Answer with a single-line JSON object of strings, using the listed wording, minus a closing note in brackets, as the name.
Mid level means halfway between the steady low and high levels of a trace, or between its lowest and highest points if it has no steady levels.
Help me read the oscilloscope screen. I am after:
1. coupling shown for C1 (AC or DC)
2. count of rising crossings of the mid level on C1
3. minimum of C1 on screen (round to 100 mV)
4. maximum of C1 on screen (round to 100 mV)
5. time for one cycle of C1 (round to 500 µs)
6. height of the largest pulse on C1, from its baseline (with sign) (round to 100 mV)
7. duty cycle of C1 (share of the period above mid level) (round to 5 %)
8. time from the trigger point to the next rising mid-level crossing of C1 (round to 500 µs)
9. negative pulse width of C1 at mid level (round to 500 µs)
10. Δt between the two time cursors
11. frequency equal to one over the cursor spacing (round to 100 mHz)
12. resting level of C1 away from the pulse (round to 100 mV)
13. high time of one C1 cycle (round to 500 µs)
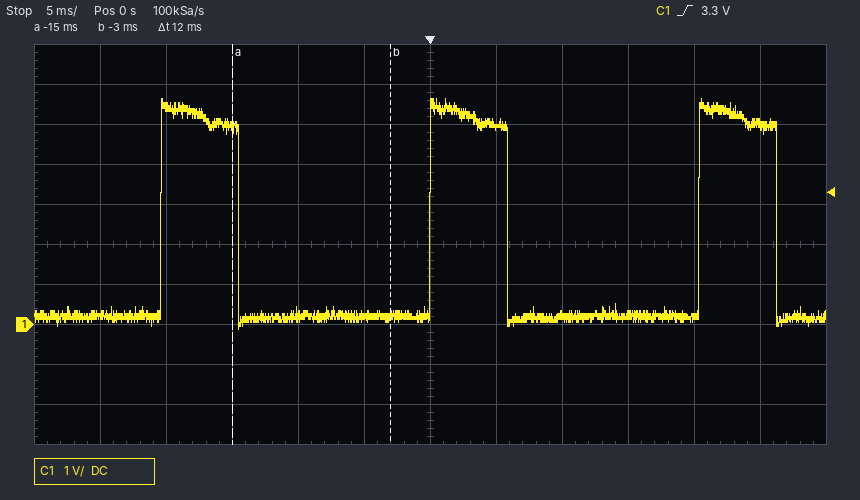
{"coupling shown for C1": "DC", "count of rising crossings of the mid level on C1": "3", "minimum of C1 on screen": "-100 mV", "maximum of C1 on screen": "5.6 V", "time for one cycle of C1": "20.5 ms", "height of the largest pulse on C1, from its baseline (with sign)": "+5.4 V", "duty cycle of C1 (share of the period above mid level)": "30 %", "time from the trigger point to the next rising mid-level crossing of C1": "20.5 ms", "negative pulse width of C1 at mid level": "14.5 ms", "Δt between the two time cursors": "12 ms", "frequency equal to one over the cursor spacing": "83.3 Hz", "resting level of C1 away from the pulse": "200 mV", "high time of one C1 cycle": "6.0 ms"}
